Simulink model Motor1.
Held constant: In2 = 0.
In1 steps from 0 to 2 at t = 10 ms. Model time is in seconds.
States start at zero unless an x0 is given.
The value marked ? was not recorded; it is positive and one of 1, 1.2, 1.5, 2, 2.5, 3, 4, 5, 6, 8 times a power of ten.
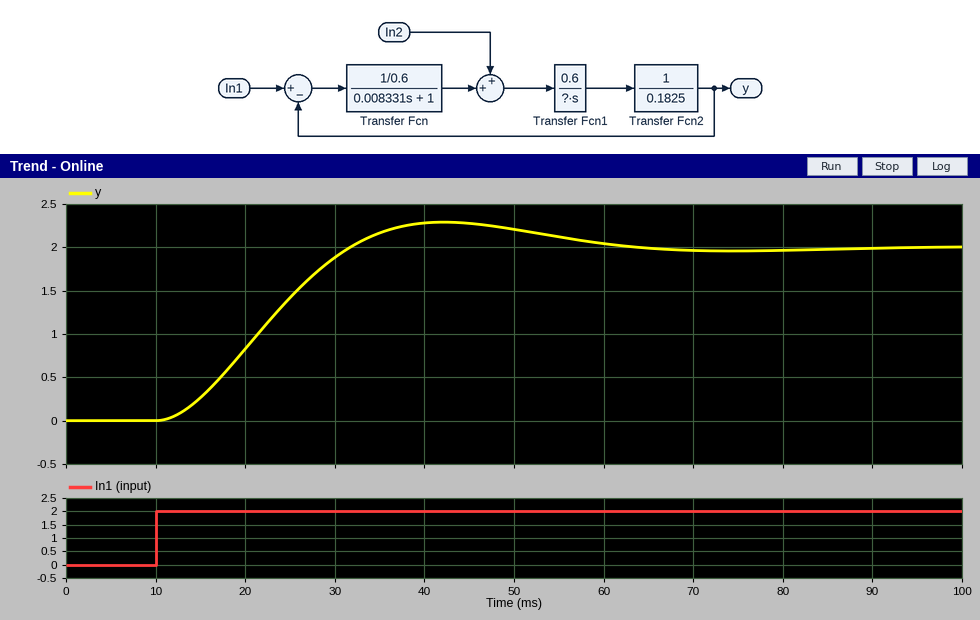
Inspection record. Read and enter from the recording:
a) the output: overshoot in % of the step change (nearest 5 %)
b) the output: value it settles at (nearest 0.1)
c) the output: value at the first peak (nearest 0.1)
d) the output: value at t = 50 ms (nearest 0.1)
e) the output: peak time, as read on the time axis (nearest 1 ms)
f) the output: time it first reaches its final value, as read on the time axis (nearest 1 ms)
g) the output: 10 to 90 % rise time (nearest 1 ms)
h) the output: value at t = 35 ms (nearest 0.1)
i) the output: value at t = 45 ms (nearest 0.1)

15 %
2.0
2.3
2.2
42 ms
32 ms
15 ms
2.2
2.3
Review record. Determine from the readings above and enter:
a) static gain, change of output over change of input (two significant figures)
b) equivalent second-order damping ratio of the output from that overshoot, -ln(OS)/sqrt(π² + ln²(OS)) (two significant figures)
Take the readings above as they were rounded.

1.0
0.52
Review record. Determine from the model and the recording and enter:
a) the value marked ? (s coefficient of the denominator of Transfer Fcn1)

0.05
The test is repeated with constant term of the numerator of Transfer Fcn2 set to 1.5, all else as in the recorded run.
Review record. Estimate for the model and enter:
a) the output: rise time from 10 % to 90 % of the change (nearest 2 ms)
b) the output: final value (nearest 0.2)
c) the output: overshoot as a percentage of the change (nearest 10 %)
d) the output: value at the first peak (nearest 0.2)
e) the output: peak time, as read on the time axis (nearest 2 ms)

10 ms
2.0
20 %
2.4
34 ms
